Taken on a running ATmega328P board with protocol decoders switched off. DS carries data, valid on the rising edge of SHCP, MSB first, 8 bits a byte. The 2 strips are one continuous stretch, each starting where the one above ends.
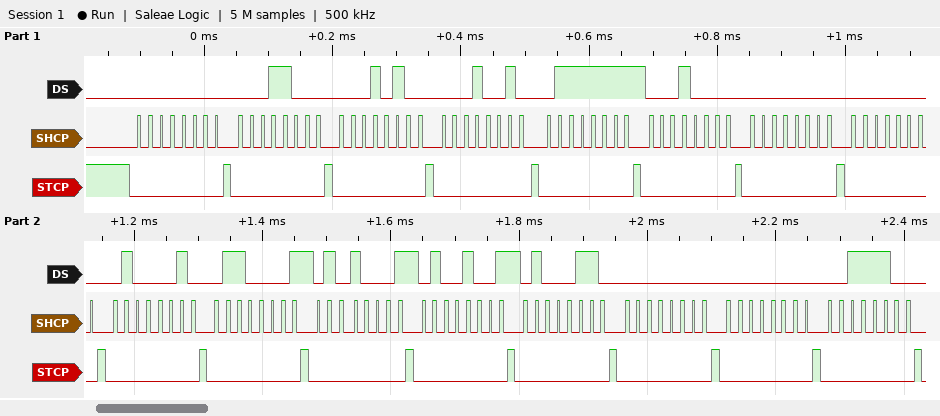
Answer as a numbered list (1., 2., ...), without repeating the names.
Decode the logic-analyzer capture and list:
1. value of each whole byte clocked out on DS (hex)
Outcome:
1. 0x00 0x18 0x14 0x12 0x7F 0x10 0x00 0x00 0x42 0x61 0x51 0x49 0x46 0x00 0x00 0x3C
